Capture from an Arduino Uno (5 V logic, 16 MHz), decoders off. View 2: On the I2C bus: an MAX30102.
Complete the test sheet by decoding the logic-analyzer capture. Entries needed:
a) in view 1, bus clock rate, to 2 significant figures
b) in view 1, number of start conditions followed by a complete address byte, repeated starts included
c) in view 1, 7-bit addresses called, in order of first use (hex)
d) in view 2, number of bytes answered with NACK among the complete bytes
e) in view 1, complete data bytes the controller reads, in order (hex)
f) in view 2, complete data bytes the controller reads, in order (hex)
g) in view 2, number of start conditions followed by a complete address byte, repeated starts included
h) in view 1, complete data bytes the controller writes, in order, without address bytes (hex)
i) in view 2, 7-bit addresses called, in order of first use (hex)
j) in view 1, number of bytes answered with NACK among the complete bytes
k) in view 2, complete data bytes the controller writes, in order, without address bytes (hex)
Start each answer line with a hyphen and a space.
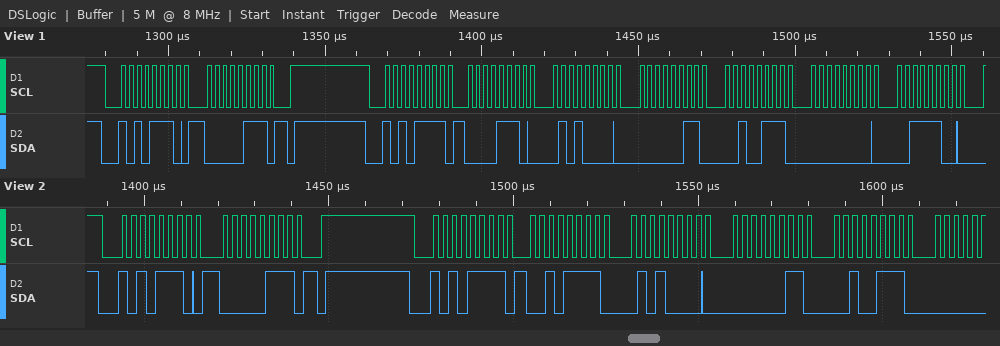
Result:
- 400 kHz
- 2
- 0x57
- 0
- 0E 50 03 27 00 3C
- 2F 50 03 27
- 2
- 07
- 0x57
- 0
- 07
